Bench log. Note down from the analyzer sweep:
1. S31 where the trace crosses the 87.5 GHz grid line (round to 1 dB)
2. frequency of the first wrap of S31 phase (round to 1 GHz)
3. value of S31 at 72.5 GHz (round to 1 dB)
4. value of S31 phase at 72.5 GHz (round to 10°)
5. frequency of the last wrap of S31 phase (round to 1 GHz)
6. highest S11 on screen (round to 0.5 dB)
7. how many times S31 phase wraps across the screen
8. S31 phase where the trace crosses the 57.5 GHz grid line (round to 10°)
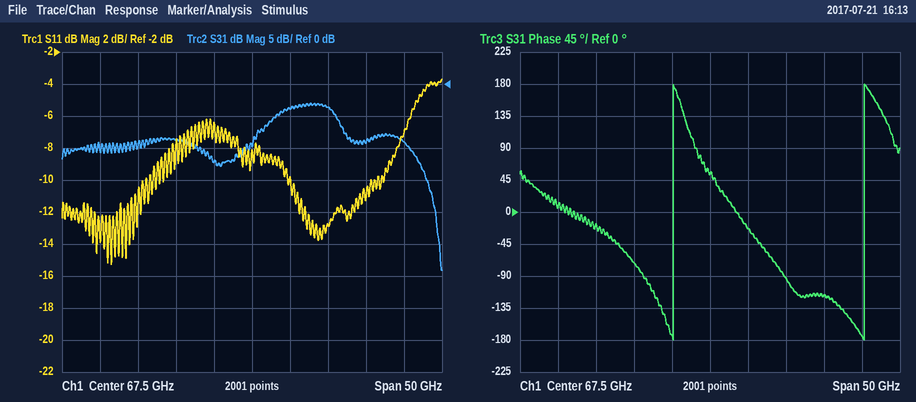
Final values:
-9 dB
63 GHz
-4 dB
-20°
88 GHz
-3.5 dB
2
-70°
